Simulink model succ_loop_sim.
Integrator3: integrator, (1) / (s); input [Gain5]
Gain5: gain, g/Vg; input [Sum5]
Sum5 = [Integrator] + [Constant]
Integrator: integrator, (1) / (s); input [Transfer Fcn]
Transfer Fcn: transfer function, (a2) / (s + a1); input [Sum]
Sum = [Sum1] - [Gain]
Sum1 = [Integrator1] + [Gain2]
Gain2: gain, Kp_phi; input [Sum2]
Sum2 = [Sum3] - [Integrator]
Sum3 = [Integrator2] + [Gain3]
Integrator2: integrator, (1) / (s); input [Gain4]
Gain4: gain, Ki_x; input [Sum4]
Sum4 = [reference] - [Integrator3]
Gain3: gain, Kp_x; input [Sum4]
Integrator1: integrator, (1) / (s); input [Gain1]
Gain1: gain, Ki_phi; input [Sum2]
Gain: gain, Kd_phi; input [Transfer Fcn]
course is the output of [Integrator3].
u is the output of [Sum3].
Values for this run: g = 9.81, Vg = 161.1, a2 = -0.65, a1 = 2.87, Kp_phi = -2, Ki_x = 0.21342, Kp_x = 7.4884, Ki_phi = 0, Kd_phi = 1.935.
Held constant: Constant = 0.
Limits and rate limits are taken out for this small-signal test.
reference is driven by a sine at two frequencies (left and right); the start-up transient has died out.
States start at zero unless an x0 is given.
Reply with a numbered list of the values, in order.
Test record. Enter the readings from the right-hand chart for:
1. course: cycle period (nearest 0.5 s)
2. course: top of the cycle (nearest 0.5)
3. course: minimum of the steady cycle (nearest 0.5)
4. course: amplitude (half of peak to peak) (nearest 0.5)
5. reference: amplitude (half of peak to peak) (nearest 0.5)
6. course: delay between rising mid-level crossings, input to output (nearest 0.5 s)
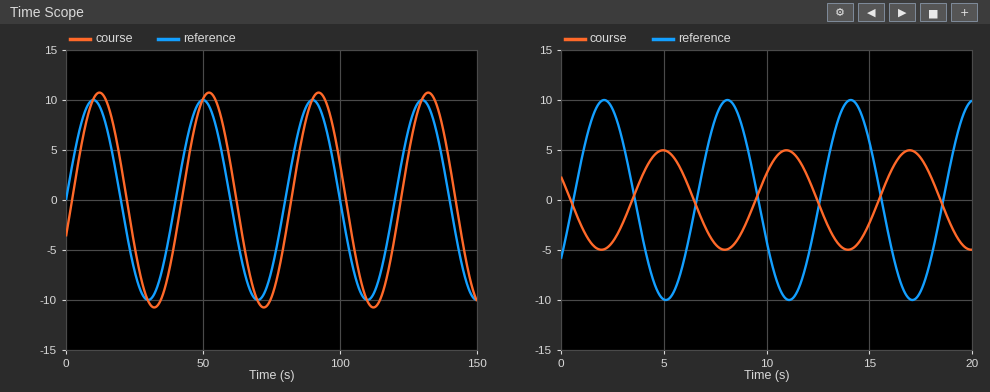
1. 6.0 s
2. 5.0
3. -5.0
4. 5.0
5. 10.0
6. 3.0 s
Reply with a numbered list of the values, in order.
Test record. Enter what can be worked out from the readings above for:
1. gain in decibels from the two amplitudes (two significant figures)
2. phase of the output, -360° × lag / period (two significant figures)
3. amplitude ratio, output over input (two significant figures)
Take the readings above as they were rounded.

1. -6.0 dB
2. -180°
3. 0.50
